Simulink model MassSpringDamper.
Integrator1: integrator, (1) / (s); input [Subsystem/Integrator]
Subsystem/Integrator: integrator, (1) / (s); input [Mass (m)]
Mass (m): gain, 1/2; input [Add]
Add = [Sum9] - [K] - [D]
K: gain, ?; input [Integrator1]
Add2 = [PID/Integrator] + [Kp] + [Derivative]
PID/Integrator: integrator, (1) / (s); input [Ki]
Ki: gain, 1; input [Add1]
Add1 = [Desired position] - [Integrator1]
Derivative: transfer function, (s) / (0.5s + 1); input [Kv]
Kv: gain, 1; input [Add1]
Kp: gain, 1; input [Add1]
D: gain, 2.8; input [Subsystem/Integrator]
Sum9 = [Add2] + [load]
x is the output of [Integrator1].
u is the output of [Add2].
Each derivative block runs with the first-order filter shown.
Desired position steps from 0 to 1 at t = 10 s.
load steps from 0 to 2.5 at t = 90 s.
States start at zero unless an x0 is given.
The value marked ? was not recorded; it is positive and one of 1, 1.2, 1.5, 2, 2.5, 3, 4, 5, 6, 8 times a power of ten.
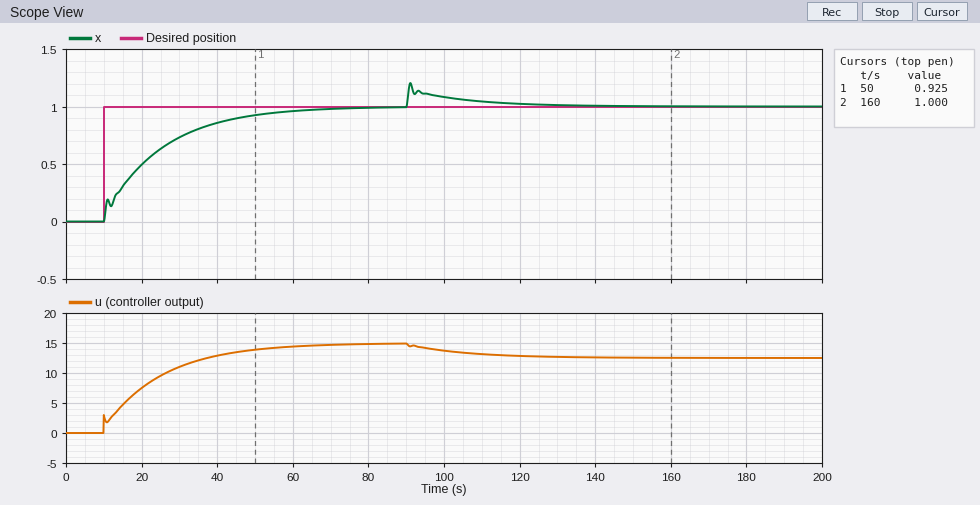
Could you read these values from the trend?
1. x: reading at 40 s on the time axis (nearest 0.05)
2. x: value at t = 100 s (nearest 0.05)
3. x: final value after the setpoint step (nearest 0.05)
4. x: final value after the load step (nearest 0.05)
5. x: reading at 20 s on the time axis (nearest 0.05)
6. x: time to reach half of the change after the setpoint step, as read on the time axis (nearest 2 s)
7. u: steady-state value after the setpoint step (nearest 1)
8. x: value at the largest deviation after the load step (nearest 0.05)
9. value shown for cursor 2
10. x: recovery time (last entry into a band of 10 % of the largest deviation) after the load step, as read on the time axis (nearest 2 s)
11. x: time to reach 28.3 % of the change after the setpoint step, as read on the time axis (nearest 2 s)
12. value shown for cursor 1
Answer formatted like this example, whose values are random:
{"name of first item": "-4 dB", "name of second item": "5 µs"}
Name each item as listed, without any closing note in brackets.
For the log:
{"x: reading at 40 s on the time axis": "0.85", "x: value at t = 100 s": "1.10", "x: final value after the setpoint step": "1.00", "x: final value after the load step": "1.00", "x: reading at 20 s on the time axis": "0.50", "x: time to reach half of the change after the setpoint step, as read on the time axis": "20 s", "u: steady-state value after the setpoint step": "15", "x: value at the largest deviation after the load step": "1.20", "value shown for cursor 2": "1.000", "x: recovery time (last entry into a band of 10 % of the largest deviation) after the load step, as read on the time axis": "122 s", "x: time to reach 28.3 % of the change after the setpoint step, as read on the time axis": "14 s", "value shown for cursor 1": "0.925"}
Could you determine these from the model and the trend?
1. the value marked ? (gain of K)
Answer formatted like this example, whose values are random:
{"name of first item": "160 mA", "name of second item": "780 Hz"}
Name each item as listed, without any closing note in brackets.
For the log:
{"the value marked ?": "15"}
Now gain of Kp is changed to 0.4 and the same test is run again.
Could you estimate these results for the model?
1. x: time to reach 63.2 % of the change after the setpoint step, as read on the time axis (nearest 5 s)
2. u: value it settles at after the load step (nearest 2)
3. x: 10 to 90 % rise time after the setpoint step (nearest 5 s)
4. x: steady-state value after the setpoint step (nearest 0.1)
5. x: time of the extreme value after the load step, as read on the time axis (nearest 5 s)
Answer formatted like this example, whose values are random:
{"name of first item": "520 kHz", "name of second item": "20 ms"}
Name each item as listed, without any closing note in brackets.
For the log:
{"x: time to reach 63.2 % of the change after the setpoint step, as read on the time axis": "25 s", "u: value it settles at after the load step": "12", "x: 10 to 90 % rise time after the setpoint step": "35 s", "x: steady-state value after the setpoint step": "1.0", "x: time of the extreme value after the load step, as read on the time axis": "90 s"}
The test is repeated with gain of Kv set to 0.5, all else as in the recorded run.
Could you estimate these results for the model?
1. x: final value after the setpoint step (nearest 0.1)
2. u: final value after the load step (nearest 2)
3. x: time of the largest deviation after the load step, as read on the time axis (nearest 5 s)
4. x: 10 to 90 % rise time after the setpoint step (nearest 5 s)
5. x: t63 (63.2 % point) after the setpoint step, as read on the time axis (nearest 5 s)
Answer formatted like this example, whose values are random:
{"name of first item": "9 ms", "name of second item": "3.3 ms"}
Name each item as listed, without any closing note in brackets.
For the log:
{"x: final value after the setpoint step": "1.0", "u: final value after the load step": "12", "x: time of the largest deviation after the load step, as read on the time axis": "90 s", "x: 10 to 90 % rise time after the setpoint step": "35 s", "x: t63 (63.2 % point) after the setpoint step, as read on the time axis": "25 s"}
